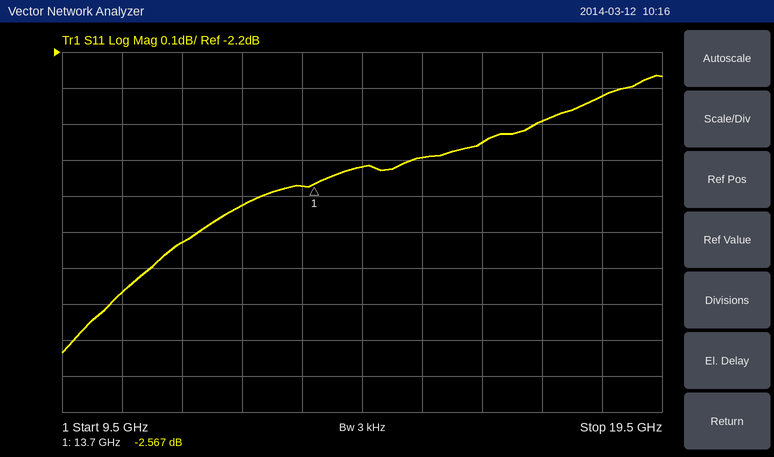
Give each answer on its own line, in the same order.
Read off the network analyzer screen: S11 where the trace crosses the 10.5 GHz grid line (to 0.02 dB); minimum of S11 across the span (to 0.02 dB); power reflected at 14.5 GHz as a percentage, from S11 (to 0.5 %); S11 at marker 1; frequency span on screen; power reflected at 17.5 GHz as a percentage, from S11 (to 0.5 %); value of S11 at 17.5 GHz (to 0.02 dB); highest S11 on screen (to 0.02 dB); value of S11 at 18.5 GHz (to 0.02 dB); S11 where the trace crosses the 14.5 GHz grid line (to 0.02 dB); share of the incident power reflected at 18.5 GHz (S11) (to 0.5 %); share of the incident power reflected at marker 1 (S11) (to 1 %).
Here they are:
-2.86 dB
-3.04 dB
56.0 %
-2.567 dB
10 GHz
57.5 %
-2.40 dB
-2.26 dB
-2.32 dB
-2.52 dB
58.5 %
55 %
